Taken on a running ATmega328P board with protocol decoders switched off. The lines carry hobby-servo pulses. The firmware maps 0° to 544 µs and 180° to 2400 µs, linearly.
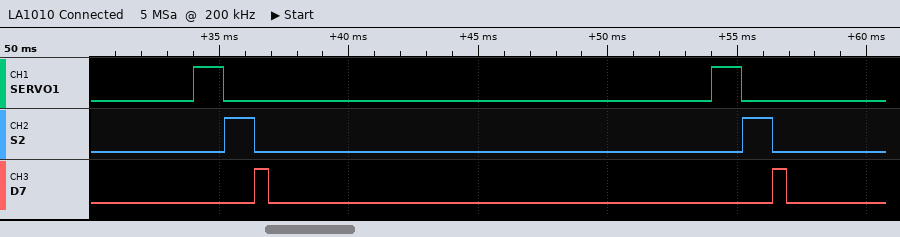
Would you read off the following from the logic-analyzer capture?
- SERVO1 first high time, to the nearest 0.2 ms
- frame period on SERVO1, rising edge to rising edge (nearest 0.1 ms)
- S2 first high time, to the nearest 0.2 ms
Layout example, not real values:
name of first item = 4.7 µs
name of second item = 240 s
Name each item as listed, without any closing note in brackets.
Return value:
SERVO1 first high time, to the nearest 0.2 ms = 1.2 ms
frame period on SERVO1, rising edge to rising edge = 20.0 ms
S2 first high time, to the nearest 0.2 ms = 1.2 ms
